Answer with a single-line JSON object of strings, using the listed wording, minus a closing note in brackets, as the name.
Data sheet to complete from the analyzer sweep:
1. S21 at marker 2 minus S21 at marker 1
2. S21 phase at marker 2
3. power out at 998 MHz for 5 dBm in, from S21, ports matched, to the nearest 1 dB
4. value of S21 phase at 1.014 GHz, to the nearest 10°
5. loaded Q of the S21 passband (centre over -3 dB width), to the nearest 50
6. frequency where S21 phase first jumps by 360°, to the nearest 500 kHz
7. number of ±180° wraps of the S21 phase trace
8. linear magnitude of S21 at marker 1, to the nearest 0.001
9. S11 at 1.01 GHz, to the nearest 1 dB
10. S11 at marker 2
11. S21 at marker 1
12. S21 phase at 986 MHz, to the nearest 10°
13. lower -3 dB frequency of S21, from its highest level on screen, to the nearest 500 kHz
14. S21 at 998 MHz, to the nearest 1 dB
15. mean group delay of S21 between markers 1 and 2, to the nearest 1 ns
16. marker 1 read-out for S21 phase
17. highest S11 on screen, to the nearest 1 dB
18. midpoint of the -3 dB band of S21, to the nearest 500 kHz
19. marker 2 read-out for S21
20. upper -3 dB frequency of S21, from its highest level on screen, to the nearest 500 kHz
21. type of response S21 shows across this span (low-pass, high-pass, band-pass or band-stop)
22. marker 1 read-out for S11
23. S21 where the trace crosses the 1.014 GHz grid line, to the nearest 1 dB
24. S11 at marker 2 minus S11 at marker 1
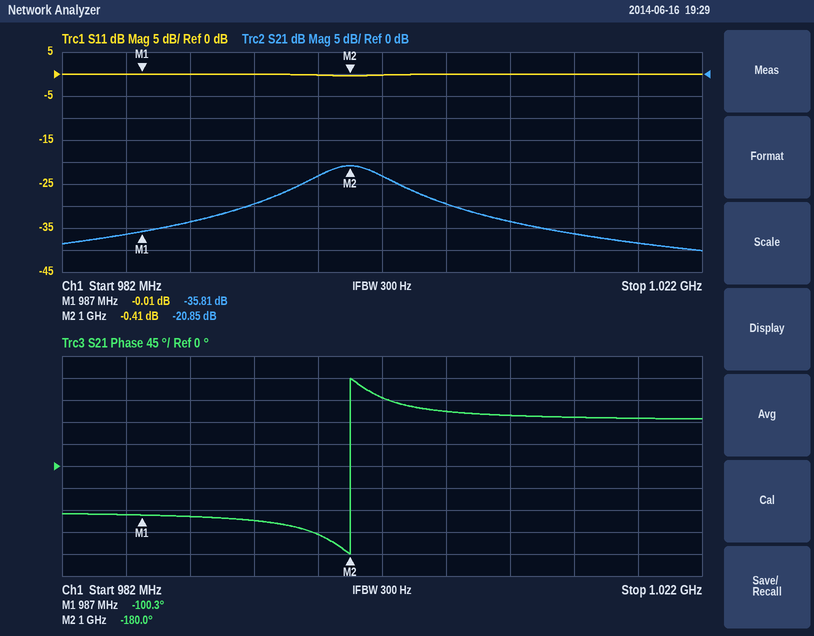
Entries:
{"S21 at marker 2 minus S21 at marker 1": "14.96 dB", "S21 phase at marker 2": "-180.0°", "power out at 998 MHz for 5 dBm in, from S21, ports matched, to the nearest 1 dB": "-18 dBm", "value of S21 phase at 1.014 GHz, to the nearest 10°": "100°", "loaded Q of the S21 passband (centre over -3 dB width), to the nearest 50": "200", "frequency where S21 phase first jumps by 360°, to the nearest 500 kHz": "1.0000 GHz", "number of ±180° wraps of the S21 phase trace": "1", "linear magnitude of S21 at marker 1, to the nearest 0.001": "0.016", "S11 at 1.01 GHz, to the nearest 1 dB": "0 dB", "S11 at marker 2": "-0.41 dB", "S21 at marker 1": "-35.81 dB", "S21 phase at 986 MHz, to the nearest 10°": "-100°", "lower -3 dB frequency of S21, from its highest level on screen, to the nearest 500 kHz": "997.5 MHz", "S21 at 998 MHz, to the nearest 1 dB": "-23 dB", "mean group delay of S21 between markers 1 and 2, to the nearest 1 ns": "17 ns", "marker 1 read-out for S21 phase": "-100.3°", "highest S11 on screen, to the nearest 1 dB": "0 dB", "midpoint of the -3 dB band of S21, to the nearest 500 kHz": "1.0000 GHz", "marker 2 read-out for S21": "-20.85 dB", "upper -3 dB frequency of S21, from its highest level on screen, to the nearest 500 kHz": "1.0025 GHz", "type of response S21 shows across this span": "band-pass", "marker 1 read-out for S11": "-0.01 dB", "S21 where the trace crosses the 1.014 GHz grid line, to the nearest 1 dB": "-36 dB", "S11 at marker 2 minus S11 at marker 1": "-0.40 dB"}
